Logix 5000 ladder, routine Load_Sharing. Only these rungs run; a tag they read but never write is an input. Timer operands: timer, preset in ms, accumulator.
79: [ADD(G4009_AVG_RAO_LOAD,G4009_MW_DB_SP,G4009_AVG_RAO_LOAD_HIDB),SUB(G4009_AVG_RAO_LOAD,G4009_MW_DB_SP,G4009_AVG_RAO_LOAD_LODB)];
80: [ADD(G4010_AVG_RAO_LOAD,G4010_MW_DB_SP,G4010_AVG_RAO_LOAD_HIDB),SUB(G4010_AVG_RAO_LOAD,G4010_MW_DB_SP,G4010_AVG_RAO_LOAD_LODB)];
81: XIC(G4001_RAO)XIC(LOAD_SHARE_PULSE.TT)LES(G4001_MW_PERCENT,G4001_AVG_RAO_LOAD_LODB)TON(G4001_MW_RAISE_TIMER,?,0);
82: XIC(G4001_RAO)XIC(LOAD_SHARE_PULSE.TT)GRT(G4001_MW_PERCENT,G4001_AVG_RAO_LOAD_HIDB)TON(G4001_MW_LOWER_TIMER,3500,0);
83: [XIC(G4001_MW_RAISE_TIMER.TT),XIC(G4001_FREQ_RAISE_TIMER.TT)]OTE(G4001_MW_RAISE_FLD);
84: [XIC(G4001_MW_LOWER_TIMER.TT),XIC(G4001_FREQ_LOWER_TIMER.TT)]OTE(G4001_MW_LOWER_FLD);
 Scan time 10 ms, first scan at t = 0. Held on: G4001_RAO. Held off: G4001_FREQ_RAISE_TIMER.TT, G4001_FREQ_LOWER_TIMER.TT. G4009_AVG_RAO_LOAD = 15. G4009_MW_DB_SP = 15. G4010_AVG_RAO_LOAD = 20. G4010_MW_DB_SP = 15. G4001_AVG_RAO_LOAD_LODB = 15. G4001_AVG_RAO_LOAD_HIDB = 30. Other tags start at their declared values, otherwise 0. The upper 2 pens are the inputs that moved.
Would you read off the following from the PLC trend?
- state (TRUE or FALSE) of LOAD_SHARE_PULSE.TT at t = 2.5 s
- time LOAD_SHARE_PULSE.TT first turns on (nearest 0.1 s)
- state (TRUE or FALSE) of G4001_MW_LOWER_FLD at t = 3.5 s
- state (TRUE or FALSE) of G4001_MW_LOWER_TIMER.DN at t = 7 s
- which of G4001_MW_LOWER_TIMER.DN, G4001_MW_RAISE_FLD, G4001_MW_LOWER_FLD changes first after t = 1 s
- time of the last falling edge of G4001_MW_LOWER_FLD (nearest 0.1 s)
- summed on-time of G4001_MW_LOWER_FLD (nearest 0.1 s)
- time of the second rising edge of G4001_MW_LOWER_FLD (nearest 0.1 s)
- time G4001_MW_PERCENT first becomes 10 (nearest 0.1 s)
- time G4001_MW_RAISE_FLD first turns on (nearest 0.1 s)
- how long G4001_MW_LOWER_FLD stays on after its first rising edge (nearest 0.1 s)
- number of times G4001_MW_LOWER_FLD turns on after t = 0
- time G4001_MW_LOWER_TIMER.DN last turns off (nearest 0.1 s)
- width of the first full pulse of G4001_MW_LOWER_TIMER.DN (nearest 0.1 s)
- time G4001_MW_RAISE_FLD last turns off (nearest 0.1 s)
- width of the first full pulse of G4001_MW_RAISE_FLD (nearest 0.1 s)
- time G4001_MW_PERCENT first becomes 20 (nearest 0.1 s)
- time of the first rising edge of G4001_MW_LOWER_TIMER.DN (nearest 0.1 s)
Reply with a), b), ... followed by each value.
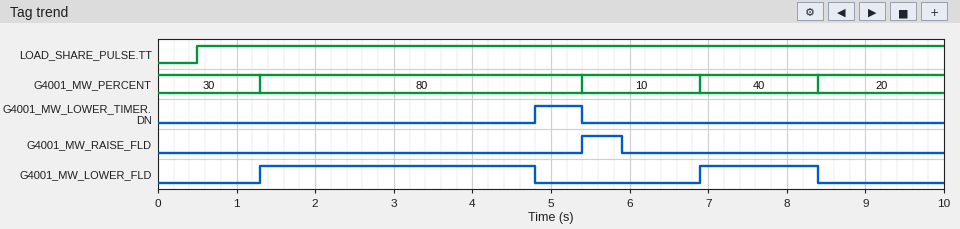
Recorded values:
a) TRUE
b) 0.5 s
c) TRUE
d) FALSE
e) G4001_MW_LOWER_FLD
f) 8.4 s
g) 5.0 s
h) 6.9 s
i) 5.4 s
j) 5.4 s
k) 3.5 s
l) 2
m) 5.4 s
n) 0.6 s
o) 5.9 s
p) 0.5 s
q) 8.4 s
r) 4.8 s
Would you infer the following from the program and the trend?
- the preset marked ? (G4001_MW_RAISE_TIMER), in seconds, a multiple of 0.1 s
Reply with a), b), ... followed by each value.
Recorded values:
a) 0.5 s
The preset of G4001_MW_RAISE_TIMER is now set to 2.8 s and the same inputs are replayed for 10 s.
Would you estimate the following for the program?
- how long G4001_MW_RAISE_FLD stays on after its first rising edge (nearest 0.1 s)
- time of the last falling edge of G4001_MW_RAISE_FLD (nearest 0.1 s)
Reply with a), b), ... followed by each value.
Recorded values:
a) 1.5 s
b) 6.9 s
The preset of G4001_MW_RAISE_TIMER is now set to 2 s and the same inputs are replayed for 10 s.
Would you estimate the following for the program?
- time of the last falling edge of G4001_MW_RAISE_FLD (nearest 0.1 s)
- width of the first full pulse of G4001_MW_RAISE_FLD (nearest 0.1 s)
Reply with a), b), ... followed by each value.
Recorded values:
a) 6.9 s
b) 1.5 s
